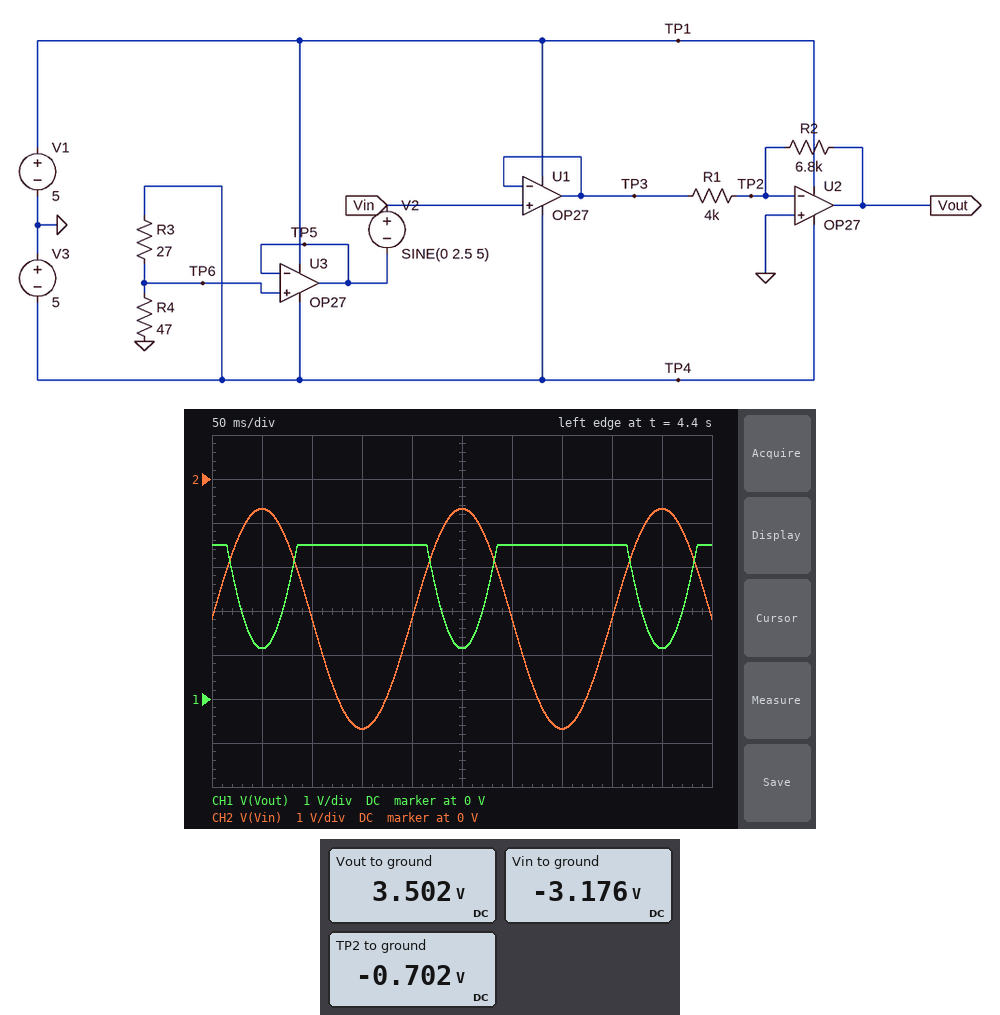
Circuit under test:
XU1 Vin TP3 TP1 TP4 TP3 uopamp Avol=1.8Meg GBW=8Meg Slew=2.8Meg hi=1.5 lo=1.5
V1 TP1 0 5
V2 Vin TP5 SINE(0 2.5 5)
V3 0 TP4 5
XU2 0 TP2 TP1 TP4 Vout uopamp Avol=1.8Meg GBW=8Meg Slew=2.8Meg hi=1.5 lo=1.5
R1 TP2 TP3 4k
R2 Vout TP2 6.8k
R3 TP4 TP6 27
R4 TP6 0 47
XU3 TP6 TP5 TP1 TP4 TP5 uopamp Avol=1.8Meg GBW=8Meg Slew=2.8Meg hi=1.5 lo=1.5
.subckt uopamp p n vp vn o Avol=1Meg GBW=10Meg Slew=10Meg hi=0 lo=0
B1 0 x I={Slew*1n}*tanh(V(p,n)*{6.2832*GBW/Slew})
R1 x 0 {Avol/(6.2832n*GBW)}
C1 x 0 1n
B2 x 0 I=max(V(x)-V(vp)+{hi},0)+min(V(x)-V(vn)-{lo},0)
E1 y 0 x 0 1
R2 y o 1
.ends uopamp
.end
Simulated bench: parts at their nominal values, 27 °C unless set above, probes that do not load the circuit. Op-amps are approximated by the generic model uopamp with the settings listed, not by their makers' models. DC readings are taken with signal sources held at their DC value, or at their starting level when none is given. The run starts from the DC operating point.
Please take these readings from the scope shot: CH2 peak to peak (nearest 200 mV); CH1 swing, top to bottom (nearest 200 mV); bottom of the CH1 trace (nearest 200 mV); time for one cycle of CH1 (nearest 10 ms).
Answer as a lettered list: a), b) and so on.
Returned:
a) 5.0 V
b) 2.4 V
c) 1.2 V
d) 200 ms
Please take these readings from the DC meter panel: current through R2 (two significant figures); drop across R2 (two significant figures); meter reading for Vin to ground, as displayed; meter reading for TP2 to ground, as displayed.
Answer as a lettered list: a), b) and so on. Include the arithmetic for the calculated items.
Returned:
a) (3.502 V - (-702 mV)) / 6.8 kΩ = 620 µA
b) 3.502 V - (-702 mV) = 4.2 V
c) -3.176 V
d) -0.702 V
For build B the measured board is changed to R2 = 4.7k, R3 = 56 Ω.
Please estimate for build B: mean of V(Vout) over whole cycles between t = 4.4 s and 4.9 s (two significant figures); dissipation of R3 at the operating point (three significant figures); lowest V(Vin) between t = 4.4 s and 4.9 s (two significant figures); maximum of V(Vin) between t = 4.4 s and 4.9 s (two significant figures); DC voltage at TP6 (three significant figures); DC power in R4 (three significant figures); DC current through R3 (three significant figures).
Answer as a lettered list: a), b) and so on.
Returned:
a) 2.1 V
b) 132 mW
c) -4.8 V
d) 220 mV
e) -2.28 V
f) 111 mW
g) 48.5 mA
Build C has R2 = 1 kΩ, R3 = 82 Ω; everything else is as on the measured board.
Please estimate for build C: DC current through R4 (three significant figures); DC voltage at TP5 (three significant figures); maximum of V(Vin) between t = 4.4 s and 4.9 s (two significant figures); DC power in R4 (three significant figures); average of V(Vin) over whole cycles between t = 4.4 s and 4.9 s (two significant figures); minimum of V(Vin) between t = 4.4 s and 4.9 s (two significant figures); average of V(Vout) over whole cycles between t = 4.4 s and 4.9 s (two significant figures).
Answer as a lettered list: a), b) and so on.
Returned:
a) 38.8 mA
b) -1.82 V
c) 680 mV
d) 70.6 mW
e) -1.8 V
f) -4.3 V
g) 420 mV
